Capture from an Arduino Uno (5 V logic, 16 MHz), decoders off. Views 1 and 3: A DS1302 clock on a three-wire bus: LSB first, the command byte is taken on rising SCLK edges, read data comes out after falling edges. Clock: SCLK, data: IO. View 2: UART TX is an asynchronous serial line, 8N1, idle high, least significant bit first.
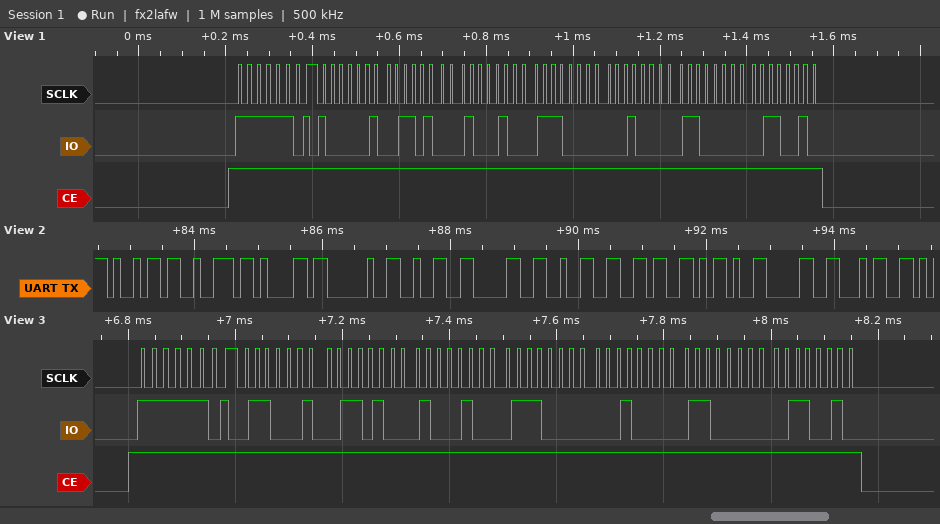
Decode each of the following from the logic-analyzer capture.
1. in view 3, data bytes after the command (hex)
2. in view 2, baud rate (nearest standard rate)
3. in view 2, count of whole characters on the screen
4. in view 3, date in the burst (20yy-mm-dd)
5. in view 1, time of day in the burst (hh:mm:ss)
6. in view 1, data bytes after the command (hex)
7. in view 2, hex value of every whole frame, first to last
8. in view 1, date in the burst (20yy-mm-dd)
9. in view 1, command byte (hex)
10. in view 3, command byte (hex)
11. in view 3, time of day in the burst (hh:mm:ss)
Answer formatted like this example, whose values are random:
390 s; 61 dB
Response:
46 16 11 07 04 03 26; 9600 baud; 11; 2026-04-07; 11:16:41; 41 16 11 07 04 03 26; 69 72 61 20 32 30 32 36 2D 30 34; 2026-04-07; 0xBF; 0xBF; 11:16:46
